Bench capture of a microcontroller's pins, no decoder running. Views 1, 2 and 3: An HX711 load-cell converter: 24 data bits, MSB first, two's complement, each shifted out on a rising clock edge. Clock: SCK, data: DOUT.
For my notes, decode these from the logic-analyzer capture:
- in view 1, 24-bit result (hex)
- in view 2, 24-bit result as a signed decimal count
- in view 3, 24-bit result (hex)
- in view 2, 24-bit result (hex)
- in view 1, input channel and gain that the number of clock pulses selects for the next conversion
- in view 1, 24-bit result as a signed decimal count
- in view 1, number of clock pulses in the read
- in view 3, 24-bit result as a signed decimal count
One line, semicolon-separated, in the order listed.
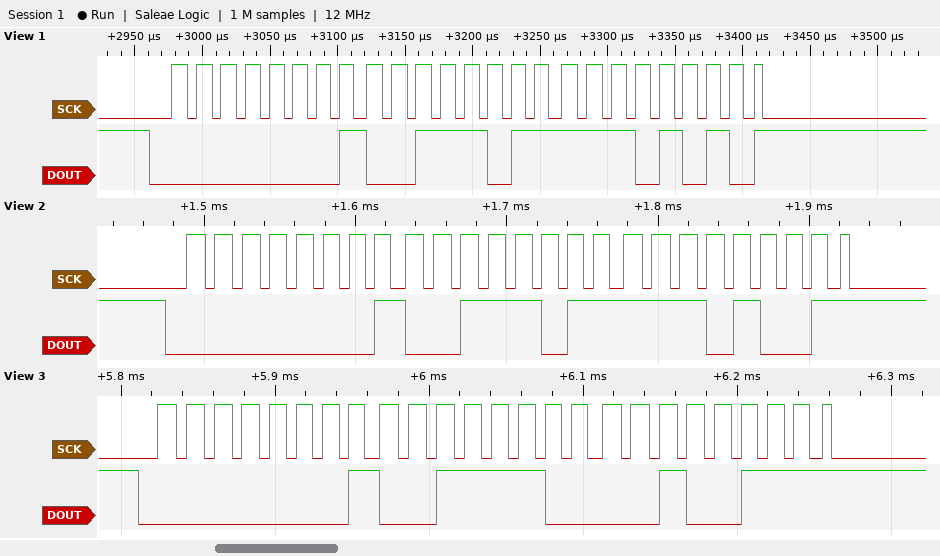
0x013BEA; 80873; 0x013C27; 0x013BE9; channel A, gain 128; 80874; 25; 80935
